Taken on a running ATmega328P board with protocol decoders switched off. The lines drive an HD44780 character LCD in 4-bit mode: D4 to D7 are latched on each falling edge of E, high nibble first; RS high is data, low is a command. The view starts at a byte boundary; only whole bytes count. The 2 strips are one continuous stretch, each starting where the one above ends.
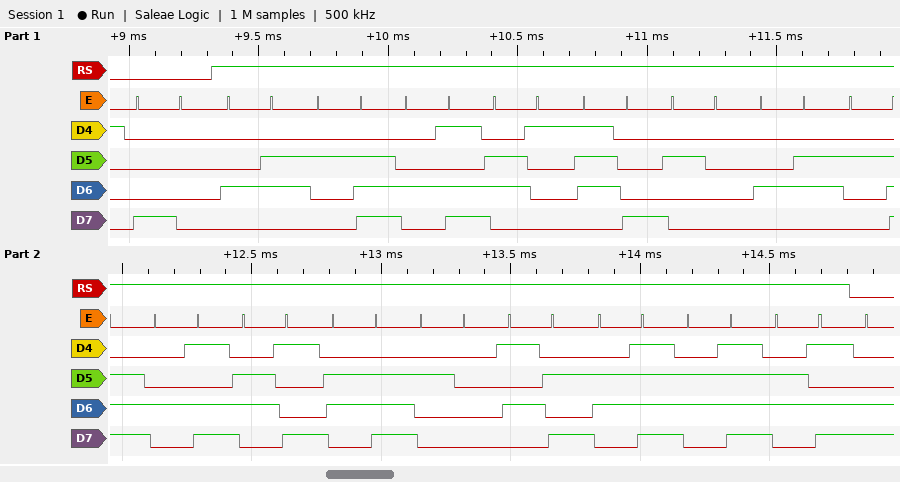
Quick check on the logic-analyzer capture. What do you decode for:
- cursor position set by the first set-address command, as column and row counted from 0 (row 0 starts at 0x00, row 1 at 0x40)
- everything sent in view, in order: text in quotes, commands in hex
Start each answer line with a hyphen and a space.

- column 0, row 0
- 0x80 "F.Max F.Min Zoom"
